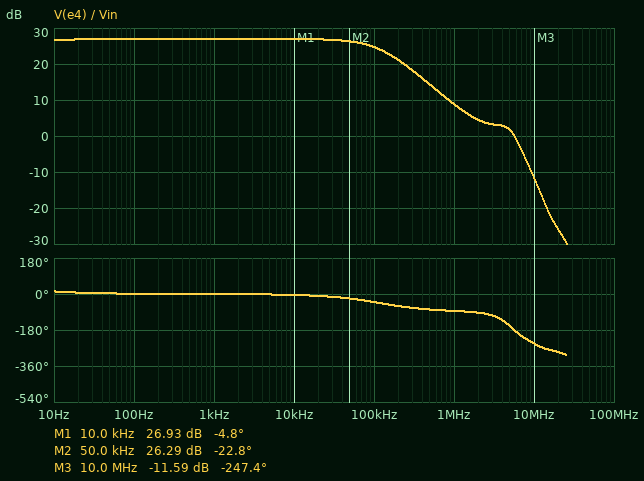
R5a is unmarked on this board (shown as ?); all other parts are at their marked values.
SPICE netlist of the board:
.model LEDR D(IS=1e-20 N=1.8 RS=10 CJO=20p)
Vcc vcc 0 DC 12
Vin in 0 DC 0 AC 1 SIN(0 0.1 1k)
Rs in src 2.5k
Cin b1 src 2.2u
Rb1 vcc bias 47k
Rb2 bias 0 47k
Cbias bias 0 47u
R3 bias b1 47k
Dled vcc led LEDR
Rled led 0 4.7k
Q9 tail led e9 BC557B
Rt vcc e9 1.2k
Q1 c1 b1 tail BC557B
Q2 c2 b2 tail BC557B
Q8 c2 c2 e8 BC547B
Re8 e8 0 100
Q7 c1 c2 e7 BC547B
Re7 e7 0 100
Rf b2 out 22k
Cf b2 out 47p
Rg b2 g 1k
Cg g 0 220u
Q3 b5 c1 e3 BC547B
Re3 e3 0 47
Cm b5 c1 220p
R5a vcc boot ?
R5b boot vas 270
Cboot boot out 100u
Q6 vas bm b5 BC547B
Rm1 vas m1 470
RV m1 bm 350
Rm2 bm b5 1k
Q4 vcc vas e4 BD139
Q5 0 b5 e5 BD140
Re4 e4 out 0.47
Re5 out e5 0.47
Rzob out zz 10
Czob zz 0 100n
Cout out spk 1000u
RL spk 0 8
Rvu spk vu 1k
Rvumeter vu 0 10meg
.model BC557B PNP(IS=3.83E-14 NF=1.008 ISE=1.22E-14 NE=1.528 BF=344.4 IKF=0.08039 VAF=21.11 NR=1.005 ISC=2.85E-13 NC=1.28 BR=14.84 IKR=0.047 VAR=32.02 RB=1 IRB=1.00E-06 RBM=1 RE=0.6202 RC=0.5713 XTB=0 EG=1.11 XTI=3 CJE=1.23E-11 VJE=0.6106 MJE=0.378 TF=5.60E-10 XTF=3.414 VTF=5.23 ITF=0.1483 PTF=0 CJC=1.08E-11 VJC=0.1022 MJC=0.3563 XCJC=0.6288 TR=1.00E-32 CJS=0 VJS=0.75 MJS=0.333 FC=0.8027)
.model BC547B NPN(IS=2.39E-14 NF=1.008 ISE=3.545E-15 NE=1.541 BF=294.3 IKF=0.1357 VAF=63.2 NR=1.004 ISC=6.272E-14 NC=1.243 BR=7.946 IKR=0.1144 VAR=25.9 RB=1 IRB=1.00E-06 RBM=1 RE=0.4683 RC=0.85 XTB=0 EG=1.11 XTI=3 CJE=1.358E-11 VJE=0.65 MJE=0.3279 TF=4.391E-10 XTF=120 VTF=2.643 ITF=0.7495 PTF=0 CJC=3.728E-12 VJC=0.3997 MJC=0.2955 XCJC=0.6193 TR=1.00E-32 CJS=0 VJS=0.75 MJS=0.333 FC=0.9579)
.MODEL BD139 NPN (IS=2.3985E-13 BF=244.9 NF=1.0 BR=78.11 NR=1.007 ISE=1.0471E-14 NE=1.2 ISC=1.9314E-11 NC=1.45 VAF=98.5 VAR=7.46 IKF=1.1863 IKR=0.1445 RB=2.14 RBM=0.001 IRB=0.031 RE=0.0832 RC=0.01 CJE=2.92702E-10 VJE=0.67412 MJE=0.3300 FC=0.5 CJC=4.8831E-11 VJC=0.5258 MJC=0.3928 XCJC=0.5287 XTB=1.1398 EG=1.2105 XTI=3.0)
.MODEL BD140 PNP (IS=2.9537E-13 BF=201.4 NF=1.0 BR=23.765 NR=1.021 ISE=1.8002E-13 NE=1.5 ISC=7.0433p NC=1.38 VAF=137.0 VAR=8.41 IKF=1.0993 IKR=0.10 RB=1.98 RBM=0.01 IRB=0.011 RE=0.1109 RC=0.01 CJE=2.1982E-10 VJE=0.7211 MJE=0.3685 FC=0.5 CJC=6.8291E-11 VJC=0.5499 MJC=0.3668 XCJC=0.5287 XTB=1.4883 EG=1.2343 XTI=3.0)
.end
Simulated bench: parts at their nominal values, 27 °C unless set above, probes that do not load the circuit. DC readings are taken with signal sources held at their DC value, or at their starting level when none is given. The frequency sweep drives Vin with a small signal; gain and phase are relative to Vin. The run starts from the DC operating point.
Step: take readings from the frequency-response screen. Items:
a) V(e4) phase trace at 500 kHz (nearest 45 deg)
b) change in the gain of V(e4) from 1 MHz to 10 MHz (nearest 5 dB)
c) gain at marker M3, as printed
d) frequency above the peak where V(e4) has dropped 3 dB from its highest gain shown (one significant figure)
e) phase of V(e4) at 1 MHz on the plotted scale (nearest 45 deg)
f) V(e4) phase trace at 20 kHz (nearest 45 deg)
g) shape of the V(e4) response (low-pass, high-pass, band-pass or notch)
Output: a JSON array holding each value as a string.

["-90 deg", "-20 dB", "-11.59 dB", "100 kHz", "-90 deg", "0 deg", "low-pass"]
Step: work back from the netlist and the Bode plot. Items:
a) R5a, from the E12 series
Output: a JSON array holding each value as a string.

["330 Ω"]
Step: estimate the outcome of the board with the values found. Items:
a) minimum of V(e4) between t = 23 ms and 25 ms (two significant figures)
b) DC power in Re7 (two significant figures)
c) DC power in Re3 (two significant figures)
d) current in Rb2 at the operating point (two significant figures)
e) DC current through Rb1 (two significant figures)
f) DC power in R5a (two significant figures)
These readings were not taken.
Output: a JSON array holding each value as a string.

["3.9 V", "26 µW", "3.7 mW", "130 µA", "130 µA", "26 mW"]
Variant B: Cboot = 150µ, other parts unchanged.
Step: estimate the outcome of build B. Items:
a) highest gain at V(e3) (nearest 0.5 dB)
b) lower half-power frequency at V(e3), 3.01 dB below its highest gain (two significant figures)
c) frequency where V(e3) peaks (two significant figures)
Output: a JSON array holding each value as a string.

["2.5 dB", "1.3 Hz", "3.2 Hz"]
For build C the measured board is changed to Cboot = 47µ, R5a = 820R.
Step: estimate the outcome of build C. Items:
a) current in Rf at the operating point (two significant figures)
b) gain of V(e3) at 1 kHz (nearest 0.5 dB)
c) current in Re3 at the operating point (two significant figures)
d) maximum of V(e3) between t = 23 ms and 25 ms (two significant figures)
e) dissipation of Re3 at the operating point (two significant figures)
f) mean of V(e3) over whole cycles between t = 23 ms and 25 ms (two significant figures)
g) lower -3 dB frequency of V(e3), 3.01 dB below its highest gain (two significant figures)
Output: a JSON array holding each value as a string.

["1.3 µA", "4.5 dB", "4.9 mA", "360 mV", "1.1 mW", "230 mV", "29 Hz"]
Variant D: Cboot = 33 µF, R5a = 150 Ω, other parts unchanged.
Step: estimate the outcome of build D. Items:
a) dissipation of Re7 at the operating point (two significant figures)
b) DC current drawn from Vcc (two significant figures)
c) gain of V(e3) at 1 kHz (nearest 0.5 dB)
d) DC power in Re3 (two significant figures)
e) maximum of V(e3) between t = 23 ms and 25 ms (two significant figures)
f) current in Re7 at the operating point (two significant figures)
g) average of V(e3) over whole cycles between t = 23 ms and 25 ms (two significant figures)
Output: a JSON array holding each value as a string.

["25 µW", "38 mA", "1.0 dB", "7.4 mW", "720 mV", "500 µA", "590 mV"]
